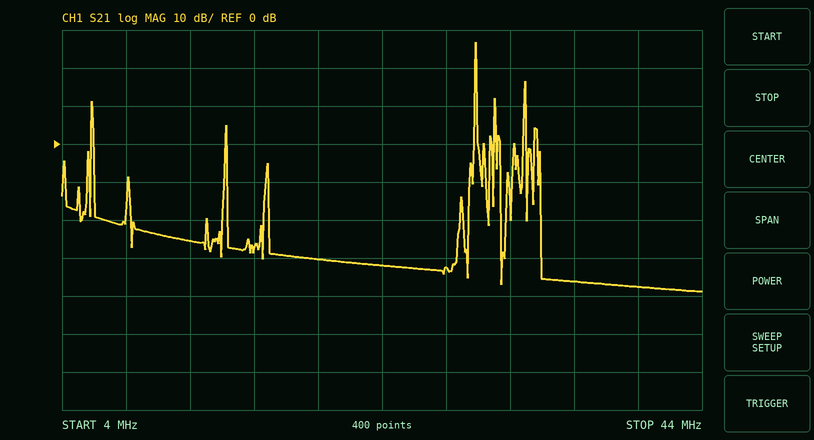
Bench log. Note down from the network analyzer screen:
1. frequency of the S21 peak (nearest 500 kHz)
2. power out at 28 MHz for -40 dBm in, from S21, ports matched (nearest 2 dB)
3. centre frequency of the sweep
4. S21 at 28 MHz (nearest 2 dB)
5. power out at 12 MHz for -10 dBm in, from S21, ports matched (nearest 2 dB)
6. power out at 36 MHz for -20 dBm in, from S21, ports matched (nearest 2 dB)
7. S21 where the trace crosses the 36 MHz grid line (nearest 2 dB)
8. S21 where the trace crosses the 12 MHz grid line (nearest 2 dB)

30.0 MHz
-72 dBm
24 MHz
-32 dB
-36 dBm
-56 dBm
-36 dB
-26 dB
